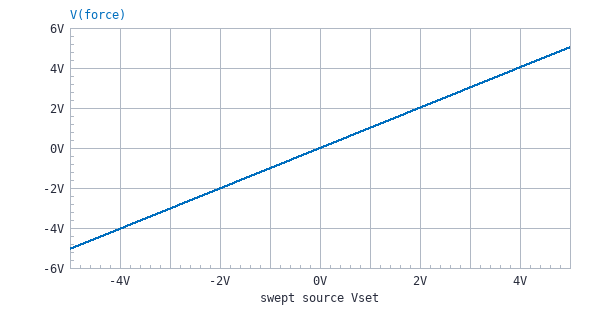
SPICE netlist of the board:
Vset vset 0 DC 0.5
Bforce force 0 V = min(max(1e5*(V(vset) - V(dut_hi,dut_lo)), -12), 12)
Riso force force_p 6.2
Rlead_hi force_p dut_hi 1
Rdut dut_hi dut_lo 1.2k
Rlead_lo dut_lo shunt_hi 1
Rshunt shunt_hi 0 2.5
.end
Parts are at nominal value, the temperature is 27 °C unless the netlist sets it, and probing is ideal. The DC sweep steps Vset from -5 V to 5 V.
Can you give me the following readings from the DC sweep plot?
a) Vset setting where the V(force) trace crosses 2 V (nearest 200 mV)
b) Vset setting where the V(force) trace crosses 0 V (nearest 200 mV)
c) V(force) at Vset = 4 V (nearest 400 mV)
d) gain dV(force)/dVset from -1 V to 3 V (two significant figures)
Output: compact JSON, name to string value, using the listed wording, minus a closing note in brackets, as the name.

{"Vset setting where the V(force) trace crosses 2 V": "2.0 V", "Vset setting where the V(force) trace crosses 0 V": "0 V", "V(force) at Vset = 4 V": "4.0 V", "gain dV(force)/dVset from -1 V to 3 V": "1.0 V/V"}
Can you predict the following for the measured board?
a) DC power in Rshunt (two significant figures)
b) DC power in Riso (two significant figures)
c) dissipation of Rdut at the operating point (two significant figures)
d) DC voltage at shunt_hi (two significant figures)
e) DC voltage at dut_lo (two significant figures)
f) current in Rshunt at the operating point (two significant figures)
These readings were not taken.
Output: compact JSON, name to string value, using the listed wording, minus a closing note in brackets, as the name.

{"DC power in Rshunt": "430 nW", "DC power in Riso": "1.1 µW", "dissipation of Rdut at the operating point": "210 µW", "DC voltage at shunt_hi": "1.0 mV", "DC voltage at dut_lo": "1.5 mV", "current in Rshunt at the operating point": "420 µA"}
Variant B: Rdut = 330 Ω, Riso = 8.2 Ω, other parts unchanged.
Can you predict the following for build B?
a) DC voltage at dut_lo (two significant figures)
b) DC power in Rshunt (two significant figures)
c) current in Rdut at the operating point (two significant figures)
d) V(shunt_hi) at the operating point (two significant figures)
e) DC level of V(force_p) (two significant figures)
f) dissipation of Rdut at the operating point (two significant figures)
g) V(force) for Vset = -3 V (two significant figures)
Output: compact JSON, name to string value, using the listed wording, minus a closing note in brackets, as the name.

{"DC voltage at dut_lo": "5.3 mV", "DC power in Rshunt": "5.7 µW", "current in Rdut at the operating point": "1.5 mA", "V(shunt_hi) at the operating point": "3.8 mV", "DC level of V(force_p)": "510 mV", "dissipation of Rdut at the operating point": "760 µW", "V(force) for Vset = -3 V": "-3.1 V"}
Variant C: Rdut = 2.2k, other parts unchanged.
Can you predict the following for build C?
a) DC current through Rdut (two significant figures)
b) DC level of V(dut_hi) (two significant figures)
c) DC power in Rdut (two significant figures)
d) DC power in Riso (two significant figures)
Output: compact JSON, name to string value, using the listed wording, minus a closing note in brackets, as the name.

{"DC current through Rdut": "230 µA", "DC level of V(dut_hi)": "500 mV", "DC power in Rdut": "110 µW", "DC power in Riso": "320 nW"}
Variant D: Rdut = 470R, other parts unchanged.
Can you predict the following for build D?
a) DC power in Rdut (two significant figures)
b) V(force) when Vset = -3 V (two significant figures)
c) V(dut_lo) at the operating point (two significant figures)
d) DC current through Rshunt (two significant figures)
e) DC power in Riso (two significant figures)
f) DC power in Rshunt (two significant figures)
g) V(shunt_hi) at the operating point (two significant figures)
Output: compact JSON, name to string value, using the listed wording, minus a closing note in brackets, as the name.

{"DC power in Rdut": "530 µW", "V(force) when Vset = -3 V": "-3.1 V", "V(dut_lo) at the operating point": "3.7 mV", "DC current through Rshunt": "1.1 mA", "DC power in Riso": "7.0 µW", "DC power in Rshunt": "2.8 µW", "V(shunt_hi) at the operating point": "2.7 mV"}
